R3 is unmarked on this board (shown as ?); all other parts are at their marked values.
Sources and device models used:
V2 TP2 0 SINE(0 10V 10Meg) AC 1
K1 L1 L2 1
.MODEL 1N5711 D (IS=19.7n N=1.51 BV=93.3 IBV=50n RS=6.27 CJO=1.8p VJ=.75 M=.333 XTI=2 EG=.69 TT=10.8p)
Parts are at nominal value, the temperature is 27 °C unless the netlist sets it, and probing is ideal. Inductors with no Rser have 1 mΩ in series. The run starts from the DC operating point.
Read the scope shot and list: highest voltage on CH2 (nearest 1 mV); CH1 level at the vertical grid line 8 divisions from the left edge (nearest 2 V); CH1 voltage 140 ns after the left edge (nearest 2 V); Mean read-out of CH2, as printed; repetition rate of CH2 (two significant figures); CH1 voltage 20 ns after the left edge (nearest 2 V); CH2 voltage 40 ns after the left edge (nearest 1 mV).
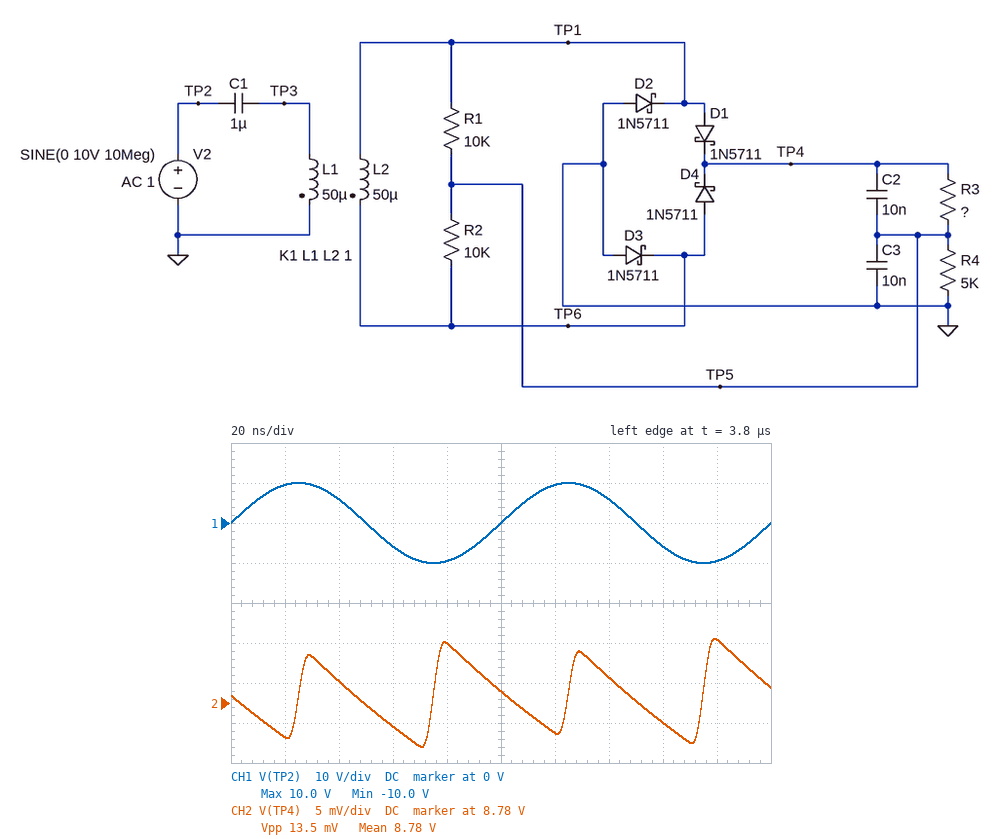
8.788 V
-6 V
6 V
8.78 V
20 MHz
10 V
8.783 V
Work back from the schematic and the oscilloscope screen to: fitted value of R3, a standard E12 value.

2.2 kΩ
